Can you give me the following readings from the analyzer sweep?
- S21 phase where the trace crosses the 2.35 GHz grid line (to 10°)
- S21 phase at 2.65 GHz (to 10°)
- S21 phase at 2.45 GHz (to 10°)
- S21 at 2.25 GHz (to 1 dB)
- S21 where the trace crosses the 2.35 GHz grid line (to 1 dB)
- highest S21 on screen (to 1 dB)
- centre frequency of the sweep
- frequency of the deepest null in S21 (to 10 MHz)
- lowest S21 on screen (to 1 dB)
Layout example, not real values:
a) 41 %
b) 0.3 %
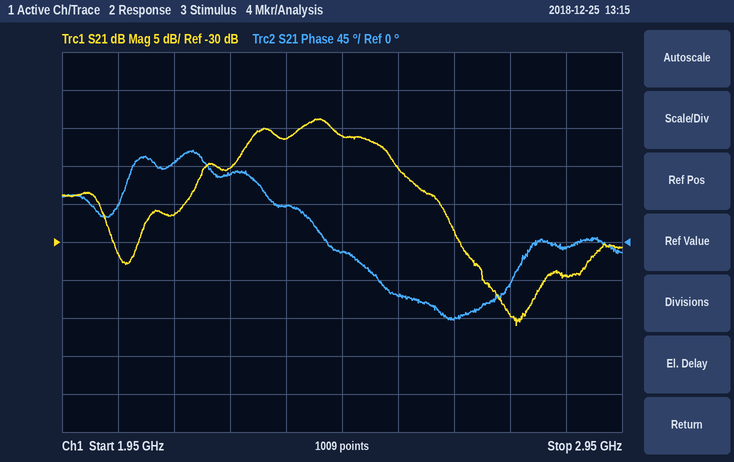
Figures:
a) 40°
b) -90°
c) -10°
d) -20 dB
e) -16 dB
f) -14 dB
g) 2.45 GHz
h) 2.76 GHz
i) -41 dB
